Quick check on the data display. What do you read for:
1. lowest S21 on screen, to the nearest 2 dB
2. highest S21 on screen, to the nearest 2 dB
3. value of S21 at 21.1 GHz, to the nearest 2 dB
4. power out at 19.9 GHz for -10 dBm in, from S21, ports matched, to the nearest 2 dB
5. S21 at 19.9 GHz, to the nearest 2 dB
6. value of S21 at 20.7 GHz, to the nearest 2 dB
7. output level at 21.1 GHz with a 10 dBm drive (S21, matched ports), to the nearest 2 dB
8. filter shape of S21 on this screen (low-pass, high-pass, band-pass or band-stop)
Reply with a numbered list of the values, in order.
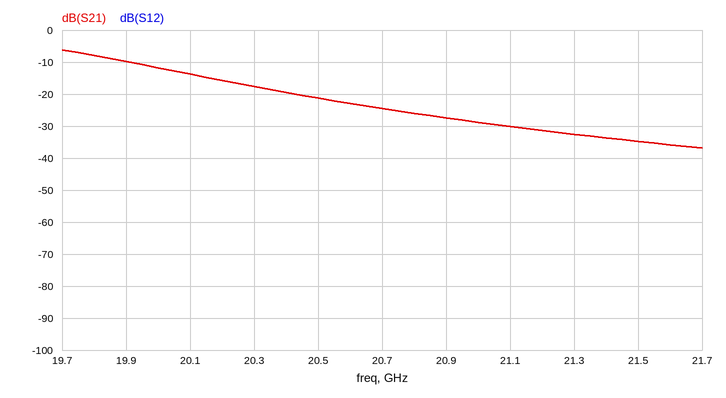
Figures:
1. -36 dB
2. -6 dB
3. -30 dB
4. -20 dBm
5. -10 dB
6. -24 dB
7. -20 dBm
8. low-pass
